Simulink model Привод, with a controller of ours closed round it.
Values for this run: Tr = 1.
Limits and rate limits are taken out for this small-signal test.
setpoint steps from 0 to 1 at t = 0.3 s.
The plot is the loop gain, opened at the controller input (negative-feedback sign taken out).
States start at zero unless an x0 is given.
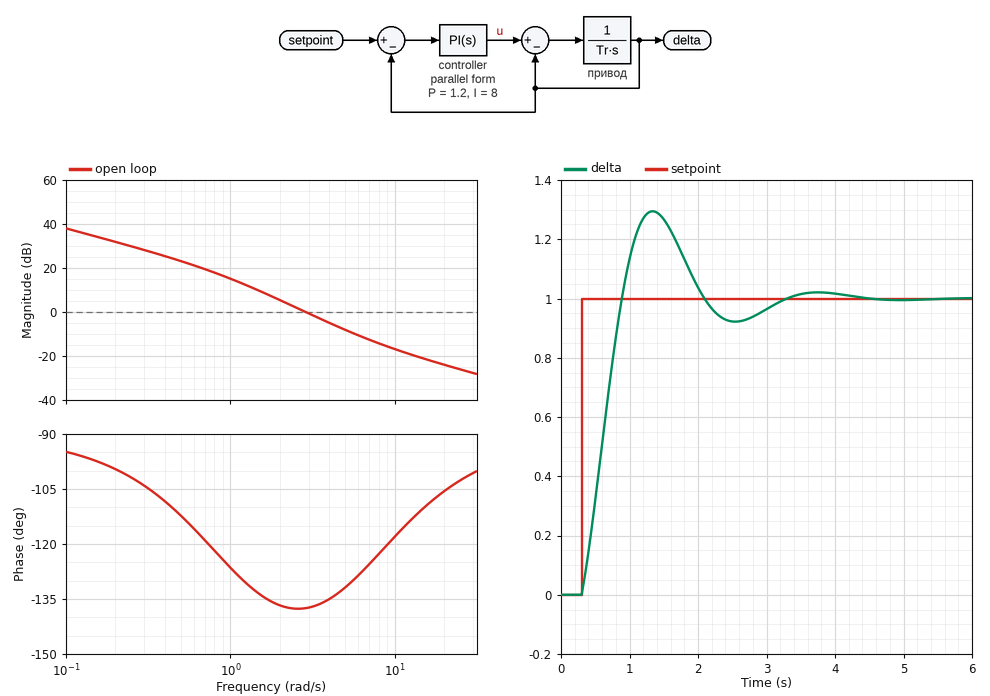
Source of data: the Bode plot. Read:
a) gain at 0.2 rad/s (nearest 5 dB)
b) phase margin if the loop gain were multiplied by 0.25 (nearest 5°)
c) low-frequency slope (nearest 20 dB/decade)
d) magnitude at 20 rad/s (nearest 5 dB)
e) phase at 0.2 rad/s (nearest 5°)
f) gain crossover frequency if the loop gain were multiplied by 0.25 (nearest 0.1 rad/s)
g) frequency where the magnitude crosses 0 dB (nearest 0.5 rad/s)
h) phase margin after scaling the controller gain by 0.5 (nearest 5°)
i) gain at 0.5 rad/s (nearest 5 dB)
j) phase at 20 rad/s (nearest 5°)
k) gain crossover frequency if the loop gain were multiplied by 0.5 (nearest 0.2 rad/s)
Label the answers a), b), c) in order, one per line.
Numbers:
a) 30 dB
b) 50°
c) -20 dB/decade
d) -25 dB
e) -100°
f) 1.3 rad/s
g) 3.0 rad/s
h) 45°
i) 25 dB
j) -105°
k) 2.0 rad/s
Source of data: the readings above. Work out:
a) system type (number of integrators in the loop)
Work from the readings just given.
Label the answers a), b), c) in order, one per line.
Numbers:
a) 1
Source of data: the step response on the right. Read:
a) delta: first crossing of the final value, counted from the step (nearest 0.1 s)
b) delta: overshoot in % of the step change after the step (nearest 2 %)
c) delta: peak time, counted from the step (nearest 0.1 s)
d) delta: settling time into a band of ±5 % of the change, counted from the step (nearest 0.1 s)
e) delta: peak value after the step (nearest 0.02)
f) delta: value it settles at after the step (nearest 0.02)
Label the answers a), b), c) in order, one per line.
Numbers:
a) 0.6 s
b) 30 %
c) 1.0 s
d) 2.6 s
e) 1.30
f) 1.00
